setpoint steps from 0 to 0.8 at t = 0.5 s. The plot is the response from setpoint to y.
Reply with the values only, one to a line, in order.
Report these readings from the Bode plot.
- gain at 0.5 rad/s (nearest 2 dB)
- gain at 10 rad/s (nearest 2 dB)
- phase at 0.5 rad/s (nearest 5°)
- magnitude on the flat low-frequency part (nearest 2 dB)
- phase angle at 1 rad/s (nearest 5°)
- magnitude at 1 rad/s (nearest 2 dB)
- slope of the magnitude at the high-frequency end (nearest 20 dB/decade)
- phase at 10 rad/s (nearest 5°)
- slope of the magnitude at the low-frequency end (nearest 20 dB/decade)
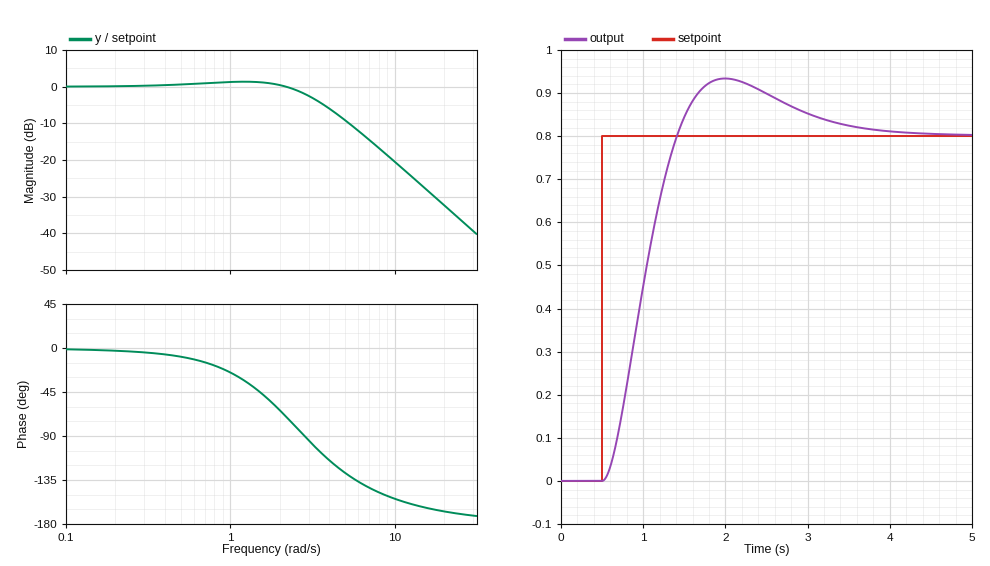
0 dB
-20 dB
-10°
0 dB
-25°
2 dB
-40 dB/decade
-155°
0 dB/decade
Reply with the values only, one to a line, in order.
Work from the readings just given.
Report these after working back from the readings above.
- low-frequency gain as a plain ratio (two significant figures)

1.0
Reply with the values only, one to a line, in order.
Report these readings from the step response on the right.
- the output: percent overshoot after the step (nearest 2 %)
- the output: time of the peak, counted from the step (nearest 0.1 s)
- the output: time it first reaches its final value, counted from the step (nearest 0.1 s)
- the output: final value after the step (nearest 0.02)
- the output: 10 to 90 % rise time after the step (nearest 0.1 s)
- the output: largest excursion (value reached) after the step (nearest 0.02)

16 %
1.5 s
0.9 s
0.80
0.6 s
0.94
